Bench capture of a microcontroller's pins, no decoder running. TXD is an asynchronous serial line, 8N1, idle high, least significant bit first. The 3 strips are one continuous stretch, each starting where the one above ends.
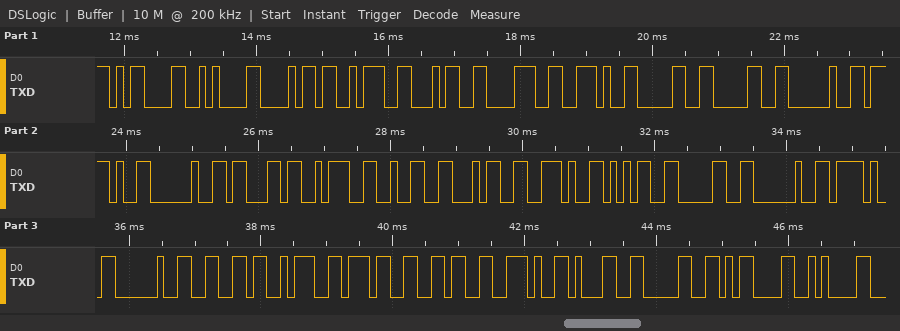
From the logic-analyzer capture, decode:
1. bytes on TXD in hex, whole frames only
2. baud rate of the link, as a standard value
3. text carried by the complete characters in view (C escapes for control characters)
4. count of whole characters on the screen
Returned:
0D 0A 68 3A 34 38 2E 30 30 20 2F 20 63 3A 32 34 2E 35 30 20 2F 20 66 3A 37 36 2E 31 30 0D 0A
9600 baud
"\r\nh:48.00 / c:24.50 / f:76.10\r\n"
31
